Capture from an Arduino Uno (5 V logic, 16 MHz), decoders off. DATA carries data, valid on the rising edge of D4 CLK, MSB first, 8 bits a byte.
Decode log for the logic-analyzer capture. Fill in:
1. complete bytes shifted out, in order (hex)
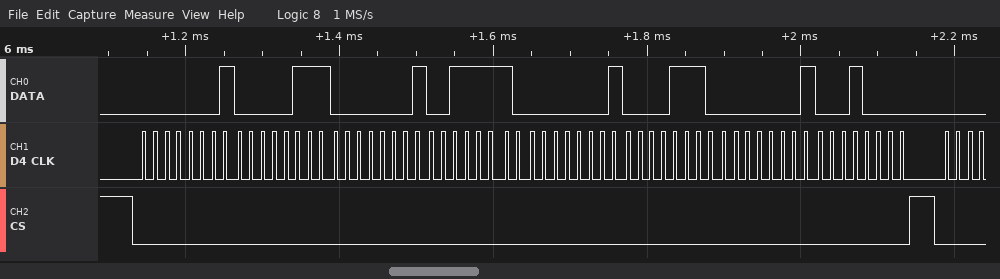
01 07 01 3E 01 0E 01 10
